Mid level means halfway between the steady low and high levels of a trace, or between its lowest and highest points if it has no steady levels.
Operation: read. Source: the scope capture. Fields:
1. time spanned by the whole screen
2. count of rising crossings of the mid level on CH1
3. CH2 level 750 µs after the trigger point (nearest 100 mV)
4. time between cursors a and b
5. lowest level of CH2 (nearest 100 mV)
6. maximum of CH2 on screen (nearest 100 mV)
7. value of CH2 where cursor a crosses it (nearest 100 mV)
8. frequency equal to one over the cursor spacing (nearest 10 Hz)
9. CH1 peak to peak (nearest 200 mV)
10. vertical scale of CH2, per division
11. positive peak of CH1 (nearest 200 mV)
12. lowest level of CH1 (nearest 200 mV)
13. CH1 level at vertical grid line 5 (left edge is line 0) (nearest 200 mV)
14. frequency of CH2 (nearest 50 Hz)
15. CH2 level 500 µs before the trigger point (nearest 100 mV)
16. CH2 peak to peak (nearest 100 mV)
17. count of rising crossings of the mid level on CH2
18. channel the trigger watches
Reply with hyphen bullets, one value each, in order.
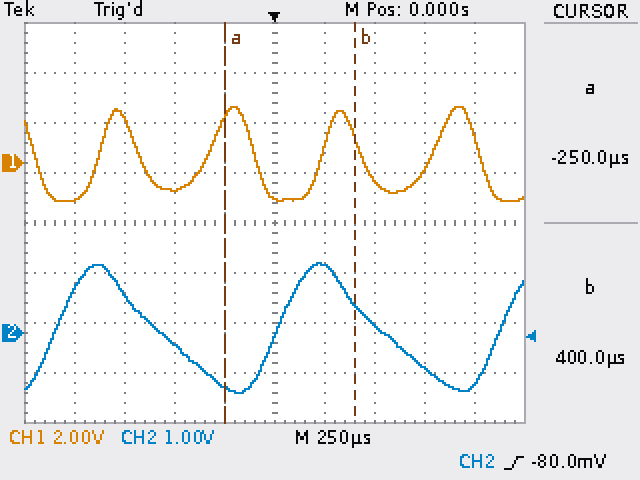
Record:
- 2.5 ms
- 4
- -700 mV
- 650 µs
- -1.2 V
- 1.4 V
- -1.1 V
- 1.54 kHz
- 3.8 V
- 1 V
- 2.2 V
- -1.6 V
- -1.4 V
- 900 Hz
- -200 mV
- 2.6 V
- 3
- CH2
